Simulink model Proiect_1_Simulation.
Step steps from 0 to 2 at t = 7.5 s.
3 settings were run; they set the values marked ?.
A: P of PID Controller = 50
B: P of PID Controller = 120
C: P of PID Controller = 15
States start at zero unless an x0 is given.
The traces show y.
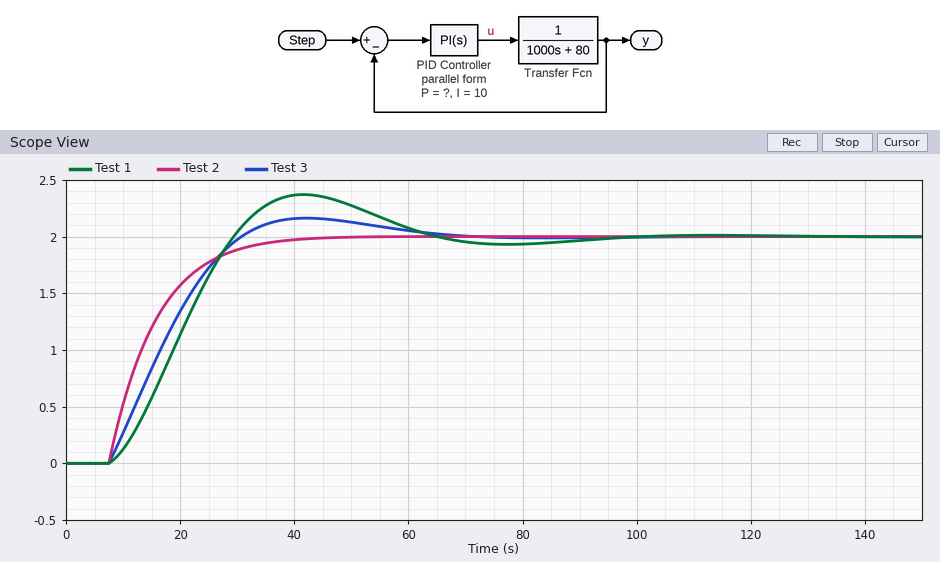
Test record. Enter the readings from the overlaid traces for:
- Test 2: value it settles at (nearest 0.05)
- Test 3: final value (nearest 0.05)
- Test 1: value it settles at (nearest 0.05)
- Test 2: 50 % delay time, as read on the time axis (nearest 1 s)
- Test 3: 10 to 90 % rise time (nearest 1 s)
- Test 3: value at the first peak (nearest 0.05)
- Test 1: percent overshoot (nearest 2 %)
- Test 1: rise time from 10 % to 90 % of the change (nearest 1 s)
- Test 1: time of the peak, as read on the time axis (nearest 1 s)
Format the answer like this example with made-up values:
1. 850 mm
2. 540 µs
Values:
1. 2.00
2. 2.00
3. 2.00
4. 13 s
5. 17 s
6. 2.15
7. 18 %
8. 16 s
9. 42 s
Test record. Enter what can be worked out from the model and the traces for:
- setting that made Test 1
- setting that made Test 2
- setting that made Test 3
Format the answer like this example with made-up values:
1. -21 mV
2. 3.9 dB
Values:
1. C
2. B
3. A
